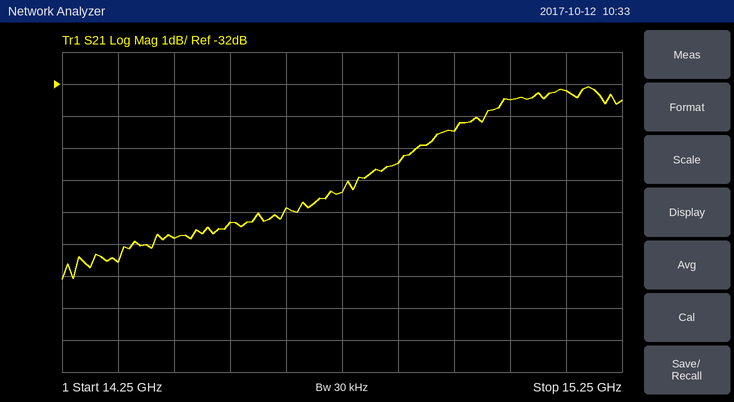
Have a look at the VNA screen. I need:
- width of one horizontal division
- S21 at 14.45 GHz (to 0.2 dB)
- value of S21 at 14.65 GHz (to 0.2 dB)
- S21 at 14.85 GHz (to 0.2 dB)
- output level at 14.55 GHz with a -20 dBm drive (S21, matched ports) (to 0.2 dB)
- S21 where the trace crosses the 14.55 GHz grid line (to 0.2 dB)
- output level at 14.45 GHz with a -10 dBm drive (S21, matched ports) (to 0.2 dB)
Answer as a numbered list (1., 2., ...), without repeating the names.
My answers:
1. 100 MHz
2. -36.8 dB
3. -35.8 dB
4. -34.4 dB
5. -56.4 dBm
6. -36.4 dB
7. -46.8 dBm
